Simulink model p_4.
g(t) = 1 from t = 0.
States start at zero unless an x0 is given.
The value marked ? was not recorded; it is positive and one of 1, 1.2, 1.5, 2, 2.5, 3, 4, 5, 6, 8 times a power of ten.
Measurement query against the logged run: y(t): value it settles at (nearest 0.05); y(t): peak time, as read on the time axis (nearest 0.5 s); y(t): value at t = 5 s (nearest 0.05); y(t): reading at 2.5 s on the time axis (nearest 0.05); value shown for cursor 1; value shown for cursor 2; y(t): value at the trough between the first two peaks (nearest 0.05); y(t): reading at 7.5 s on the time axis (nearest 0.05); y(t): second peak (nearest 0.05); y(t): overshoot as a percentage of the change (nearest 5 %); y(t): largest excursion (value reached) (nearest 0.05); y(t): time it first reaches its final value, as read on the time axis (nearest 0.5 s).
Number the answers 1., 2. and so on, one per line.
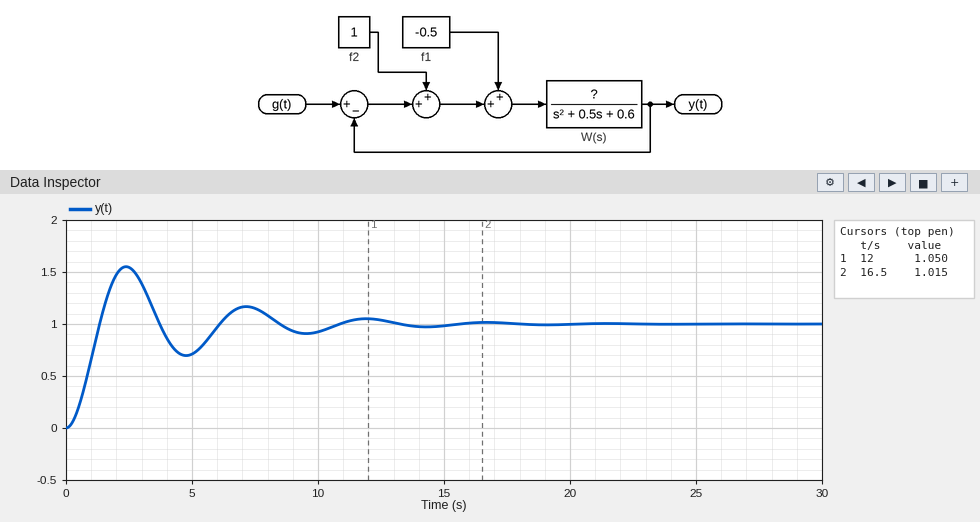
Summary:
1. 1.00
2. 2.5 s
3. 0.70
4. 1.55
5. 1.050
6. 1.015
7. 0.70
8. 1.15
9. 1.15
10. 55 %
11. 1.55
12. 1.5 s
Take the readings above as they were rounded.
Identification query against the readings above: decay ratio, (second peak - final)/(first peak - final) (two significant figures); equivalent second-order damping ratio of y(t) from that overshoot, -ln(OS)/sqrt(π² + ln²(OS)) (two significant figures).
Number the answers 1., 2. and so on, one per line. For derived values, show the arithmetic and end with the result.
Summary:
1. (1.15 - 1) / (1.55 - 1) = 0.27
2. ln(0.55) = -0.598; 0.598 / sqrt(9.870 + 0.357) = 0.19
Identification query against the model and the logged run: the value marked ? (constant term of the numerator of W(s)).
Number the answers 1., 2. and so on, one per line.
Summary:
1. 1.2
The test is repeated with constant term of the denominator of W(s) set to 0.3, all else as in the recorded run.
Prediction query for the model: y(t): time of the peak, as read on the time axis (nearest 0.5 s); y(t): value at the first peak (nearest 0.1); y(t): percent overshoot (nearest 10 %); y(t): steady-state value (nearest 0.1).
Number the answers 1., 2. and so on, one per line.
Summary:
1. 2.5 s
2. 1.8
3. 50 %
4. 1.2
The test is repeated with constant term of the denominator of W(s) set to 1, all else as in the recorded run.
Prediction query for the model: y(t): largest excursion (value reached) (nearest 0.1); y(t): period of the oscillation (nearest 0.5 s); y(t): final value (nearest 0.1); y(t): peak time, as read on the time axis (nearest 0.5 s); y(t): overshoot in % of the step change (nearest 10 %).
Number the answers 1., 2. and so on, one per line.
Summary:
1. 1.3
2. 4.5 s
3. 0.8
4. 2.0 s
5. 60 %
